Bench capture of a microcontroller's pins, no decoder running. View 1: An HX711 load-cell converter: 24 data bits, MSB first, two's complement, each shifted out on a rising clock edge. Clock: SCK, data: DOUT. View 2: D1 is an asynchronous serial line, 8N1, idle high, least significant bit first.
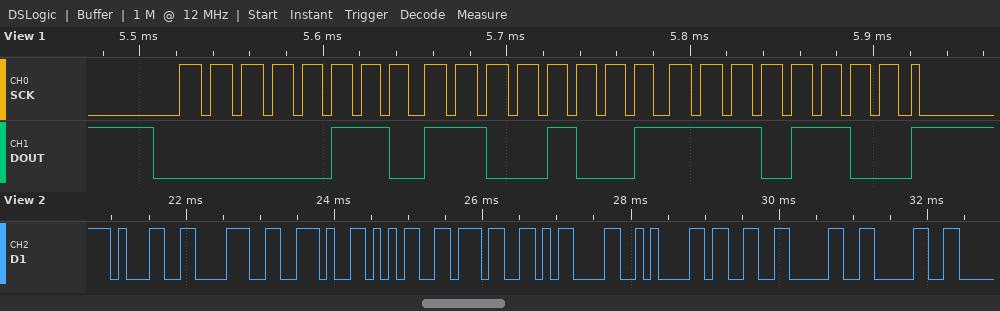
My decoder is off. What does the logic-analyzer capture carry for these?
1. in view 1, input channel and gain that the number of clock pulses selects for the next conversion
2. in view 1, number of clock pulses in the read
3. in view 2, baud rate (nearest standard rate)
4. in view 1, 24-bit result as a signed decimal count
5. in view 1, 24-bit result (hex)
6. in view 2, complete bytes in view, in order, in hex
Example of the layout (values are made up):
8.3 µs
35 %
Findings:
channel A, gain 128
25
9600 baud
444908
0x06C9EC
0x31 0x38 0x2E 0x35 0x37 0x0D 0x0A 0x33 0x30 0x30
